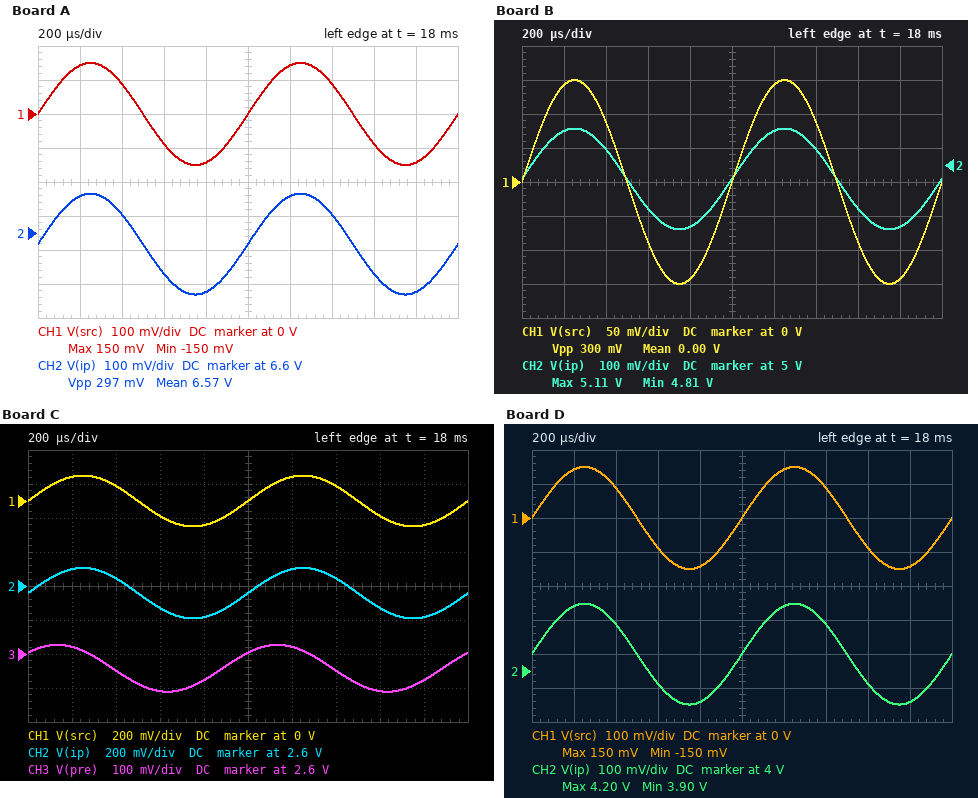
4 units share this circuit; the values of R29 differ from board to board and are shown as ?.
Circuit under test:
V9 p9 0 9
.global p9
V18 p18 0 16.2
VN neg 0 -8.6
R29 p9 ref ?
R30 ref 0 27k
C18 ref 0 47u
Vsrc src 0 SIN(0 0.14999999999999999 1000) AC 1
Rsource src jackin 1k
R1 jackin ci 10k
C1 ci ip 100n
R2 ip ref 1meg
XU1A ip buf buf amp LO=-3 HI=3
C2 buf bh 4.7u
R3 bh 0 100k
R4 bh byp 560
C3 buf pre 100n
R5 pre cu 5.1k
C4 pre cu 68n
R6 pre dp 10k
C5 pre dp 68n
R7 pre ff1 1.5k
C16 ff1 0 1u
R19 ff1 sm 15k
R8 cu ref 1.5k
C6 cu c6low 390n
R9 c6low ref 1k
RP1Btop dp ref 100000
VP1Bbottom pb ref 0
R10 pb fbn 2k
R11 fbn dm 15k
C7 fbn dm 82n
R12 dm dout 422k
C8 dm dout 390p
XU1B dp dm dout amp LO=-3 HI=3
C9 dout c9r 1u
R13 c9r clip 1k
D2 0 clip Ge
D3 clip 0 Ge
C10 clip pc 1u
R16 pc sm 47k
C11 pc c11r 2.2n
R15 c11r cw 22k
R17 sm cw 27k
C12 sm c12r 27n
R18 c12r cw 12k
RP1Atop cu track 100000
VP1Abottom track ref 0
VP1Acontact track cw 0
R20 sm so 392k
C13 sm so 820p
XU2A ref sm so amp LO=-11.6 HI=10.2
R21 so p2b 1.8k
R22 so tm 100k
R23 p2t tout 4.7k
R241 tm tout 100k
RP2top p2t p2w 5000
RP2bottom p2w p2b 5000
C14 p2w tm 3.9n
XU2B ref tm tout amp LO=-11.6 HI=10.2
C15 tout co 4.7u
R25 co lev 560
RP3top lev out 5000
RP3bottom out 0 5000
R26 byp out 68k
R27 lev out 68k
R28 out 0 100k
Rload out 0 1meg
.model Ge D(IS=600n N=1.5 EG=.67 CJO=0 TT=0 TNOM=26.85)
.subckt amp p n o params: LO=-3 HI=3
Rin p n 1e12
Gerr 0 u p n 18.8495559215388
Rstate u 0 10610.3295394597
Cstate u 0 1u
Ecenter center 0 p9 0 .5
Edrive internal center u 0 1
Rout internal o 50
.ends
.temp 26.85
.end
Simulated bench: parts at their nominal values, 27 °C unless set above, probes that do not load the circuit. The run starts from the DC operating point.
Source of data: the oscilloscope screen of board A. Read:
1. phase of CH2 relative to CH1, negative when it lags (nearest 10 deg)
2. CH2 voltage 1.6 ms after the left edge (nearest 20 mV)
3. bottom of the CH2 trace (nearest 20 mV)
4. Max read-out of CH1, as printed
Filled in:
0 deg
6.48 V
6.42 V
150 mV
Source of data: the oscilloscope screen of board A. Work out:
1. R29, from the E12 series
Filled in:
10 kΩ
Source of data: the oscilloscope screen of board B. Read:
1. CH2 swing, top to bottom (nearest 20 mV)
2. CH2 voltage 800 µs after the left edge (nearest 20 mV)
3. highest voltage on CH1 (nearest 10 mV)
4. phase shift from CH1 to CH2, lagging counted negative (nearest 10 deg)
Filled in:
300 mV
4.82 V
150 mV
0 deg
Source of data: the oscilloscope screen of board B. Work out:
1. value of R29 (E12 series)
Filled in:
22 kΩ
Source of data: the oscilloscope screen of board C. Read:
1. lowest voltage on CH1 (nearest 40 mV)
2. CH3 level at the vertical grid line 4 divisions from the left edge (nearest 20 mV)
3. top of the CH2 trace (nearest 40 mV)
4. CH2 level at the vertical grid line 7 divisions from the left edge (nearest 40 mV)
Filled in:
-160 mV
2.52 V
2.72 V
2.64 V
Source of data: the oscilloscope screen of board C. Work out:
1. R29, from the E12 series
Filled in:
68 kΩ
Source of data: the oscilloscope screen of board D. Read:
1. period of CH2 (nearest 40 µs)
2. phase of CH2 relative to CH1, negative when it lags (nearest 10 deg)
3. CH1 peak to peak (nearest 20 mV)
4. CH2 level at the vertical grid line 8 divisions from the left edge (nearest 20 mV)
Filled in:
1.00 ms
0 deg
300 mV
3.96 V
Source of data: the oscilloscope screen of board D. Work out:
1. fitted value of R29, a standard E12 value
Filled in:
33 kΩ
